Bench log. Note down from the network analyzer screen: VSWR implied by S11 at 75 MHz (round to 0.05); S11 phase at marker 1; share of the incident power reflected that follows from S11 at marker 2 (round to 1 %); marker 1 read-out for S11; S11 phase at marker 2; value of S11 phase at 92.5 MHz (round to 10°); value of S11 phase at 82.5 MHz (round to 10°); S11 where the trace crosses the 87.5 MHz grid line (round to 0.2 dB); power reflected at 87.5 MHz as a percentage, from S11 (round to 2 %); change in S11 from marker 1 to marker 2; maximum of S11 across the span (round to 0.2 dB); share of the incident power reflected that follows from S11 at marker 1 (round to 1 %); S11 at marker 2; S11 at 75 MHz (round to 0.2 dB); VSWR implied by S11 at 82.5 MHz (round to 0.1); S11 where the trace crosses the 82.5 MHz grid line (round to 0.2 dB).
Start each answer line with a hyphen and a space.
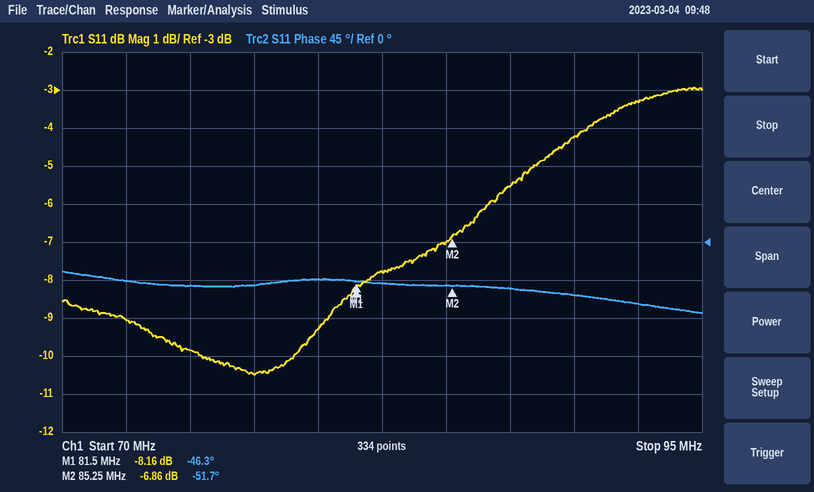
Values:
- 1.95
- -46.3°
- 21 %
- -8.16 dB
- -51.7°
- -70°
- -50°
- -5.6 dB
- 28 %
- 1.30 dB
- -3.0 dB
- 15 %
- -6.86 dB
- -9.8 dB
- 2.4
- -7.8 dB
